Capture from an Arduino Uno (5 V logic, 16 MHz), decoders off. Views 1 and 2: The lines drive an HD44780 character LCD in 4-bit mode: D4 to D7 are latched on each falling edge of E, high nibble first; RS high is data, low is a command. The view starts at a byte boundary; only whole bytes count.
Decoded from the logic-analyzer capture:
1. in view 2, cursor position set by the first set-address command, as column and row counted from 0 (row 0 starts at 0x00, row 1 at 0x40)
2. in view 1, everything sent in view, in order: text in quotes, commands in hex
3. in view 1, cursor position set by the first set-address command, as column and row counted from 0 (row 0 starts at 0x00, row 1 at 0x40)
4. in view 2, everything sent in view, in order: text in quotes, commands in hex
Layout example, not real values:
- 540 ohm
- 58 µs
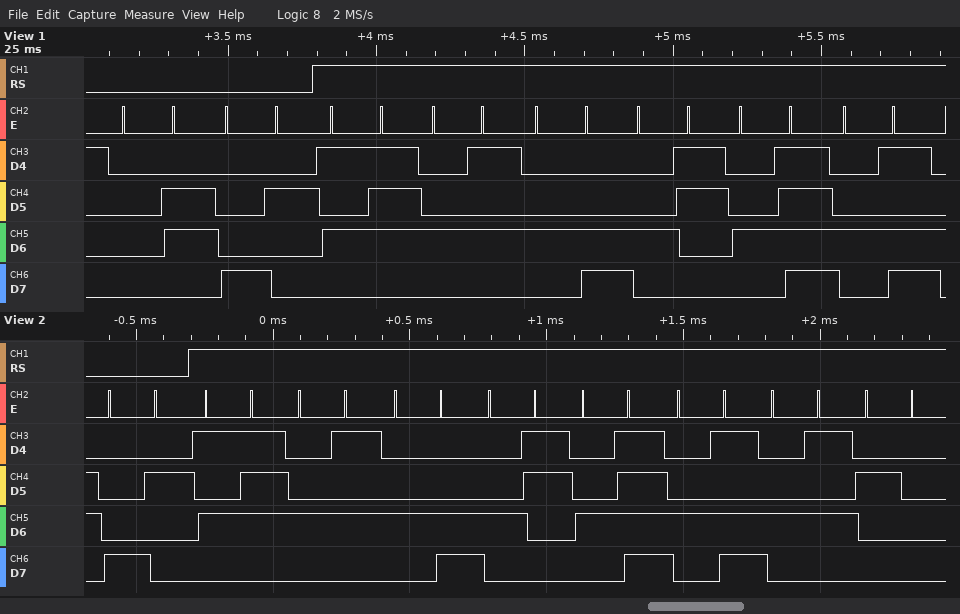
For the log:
- column 2, row 0
- 0x06 0x82 "WELCOM"
- column 2, row 0
- 0x82 "WELCOME "
